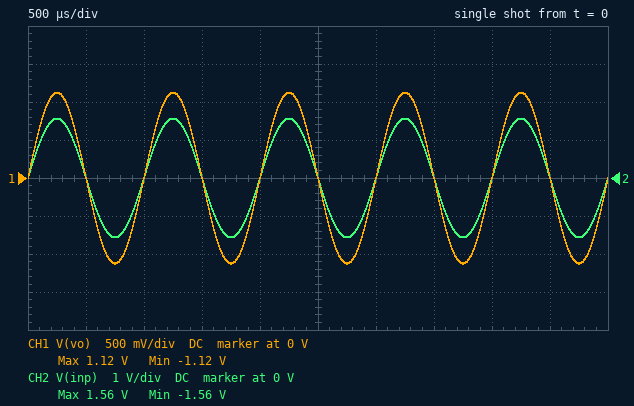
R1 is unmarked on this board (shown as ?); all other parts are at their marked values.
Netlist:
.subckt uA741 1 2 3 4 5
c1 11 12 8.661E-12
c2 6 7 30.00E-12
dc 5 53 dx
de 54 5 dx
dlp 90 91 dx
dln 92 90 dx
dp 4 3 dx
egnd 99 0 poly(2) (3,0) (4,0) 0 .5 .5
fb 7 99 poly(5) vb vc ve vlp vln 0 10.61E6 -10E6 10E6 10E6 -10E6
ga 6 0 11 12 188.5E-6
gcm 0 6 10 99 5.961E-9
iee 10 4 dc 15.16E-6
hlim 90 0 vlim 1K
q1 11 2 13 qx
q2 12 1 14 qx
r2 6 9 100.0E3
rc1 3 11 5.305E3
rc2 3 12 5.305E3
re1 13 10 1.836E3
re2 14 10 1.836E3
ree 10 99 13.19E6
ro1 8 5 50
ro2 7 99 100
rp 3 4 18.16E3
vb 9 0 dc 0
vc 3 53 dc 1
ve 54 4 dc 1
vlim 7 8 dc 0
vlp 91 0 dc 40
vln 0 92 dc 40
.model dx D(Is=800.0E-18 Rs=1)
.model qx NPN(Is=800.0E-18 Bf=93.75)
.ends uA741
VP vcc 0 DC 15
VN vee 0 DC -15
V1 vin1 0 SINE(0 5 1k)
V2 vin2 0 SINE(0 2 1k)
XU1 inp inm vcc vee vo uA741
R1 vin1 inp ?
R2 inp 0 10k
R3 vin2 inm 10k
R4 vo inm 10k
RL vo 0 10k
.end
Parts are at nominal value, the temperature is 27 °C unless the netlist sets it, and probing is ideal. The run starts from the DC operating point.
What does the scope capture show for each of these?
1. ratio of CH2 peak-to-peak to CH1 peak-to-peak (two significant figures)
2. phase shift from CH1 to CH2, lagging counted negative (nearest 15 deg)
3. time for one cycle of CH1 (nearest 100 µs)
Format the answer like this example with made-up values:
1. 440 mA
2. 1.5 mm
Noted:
1. 1.4
2. 0 deg
3. 1.0 ms
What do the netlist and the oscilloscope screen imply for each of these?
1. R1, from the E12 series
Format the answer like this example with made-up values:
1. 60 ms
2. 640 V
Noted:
1. 22 kΩ
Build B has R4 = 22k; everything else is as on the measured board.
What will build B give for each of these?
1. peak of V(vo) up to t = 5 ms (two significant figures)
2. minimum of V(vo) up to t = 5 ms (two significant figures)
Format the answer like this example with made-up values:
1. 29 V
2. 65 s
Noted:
1. 600 mV
2. -600 mV
